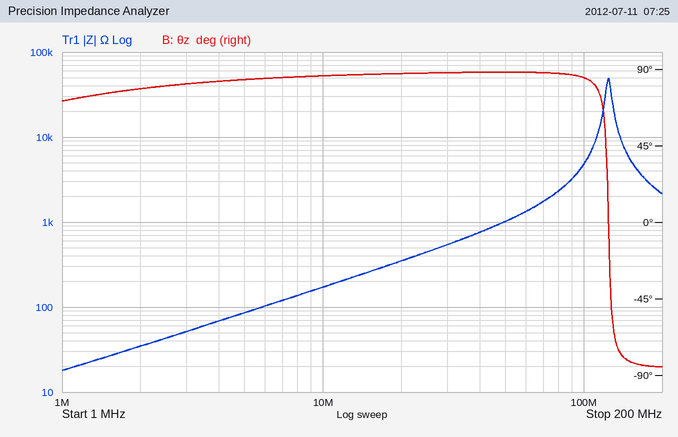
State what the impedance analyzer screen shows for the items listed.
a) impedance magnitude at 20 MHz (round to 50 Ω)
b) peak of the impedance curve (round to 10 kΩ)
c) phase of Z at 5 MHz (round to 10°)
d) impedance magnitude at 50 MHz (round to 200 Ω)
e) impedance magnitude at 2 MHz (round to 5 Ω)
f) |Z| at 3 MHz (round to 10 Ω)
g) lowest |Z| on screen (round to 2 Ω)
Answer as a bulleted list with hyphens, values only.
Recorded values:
- 350 Ω
- 50 kΩ
- 80°
- 1.0 kΩ
- 35 Ω
- 50 Ω
- 18 Ω
